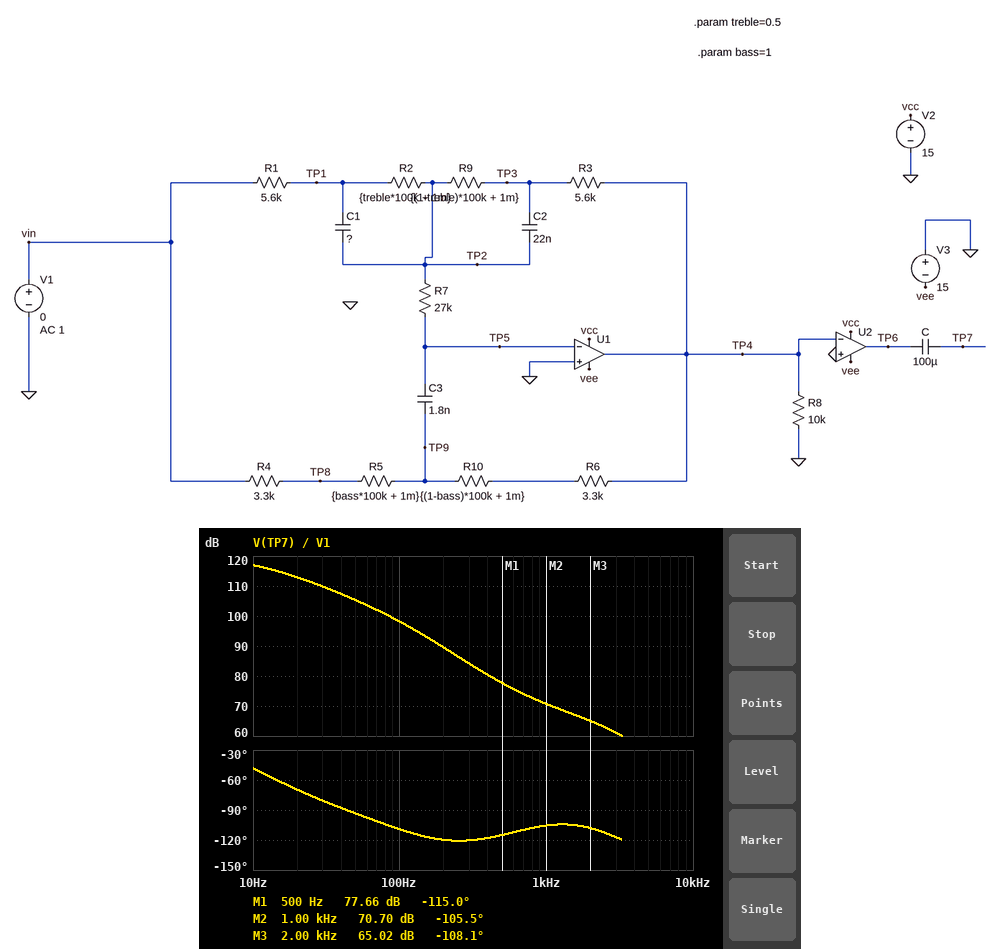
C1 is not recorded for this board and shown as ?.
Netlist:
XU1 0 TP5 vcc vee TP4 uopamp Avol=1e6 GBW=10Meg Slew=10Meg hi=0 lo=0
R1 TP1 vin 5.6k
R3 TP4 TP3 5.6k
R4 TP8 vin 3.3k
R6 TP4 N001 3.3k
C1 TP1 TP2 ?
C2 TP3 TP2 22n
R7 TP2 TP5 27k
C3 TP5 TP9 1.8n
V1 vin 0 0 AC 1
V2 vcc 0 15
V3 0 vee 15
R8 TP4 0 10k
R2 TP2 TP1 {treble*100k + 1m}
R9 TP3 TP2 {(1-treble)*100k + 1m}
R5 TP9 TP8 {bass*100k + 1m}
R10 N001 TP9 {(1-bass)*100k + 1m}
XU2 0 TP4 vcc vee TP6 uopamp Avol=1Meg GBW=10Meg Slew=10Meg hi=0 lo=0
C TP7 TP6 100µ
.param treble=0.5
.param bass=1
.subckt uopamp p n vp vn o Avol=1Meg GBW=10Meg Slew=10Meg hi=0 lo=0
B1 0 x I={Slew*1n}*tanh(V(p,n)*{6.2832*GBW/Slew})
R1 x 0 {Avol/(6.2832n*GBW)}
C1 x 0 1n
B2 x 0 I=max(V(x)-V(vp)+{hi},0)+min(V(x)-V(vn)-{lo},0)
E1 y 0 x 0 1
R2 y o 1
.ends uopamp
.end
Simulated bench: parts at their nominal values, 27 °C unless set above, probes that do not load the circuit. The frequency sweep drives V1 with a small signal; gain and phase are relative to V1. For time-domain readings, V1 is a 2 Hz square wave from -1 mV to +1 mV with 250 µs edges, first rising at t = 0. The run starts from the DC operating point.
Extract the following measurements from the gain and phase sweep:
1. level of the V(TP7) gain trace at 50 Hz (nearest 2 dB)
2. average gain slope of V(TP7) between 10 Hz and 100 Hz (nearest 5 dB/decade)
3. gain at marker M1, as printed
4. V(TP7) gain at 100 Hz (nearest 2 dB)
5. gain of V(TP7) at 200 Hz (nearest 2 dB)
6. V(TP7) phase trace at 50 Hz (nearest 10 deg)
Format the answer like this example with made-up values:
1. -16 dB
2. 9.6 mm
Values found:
1. 106 dB
2. -20 dB/decade
3. 77.66 dB
4. 98 dB
5. 90 dB
6. -90 deg
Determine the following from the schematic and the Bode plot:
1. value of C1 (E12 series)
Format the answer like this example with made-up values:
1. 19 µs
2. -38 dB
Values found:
1. 6.8 nF
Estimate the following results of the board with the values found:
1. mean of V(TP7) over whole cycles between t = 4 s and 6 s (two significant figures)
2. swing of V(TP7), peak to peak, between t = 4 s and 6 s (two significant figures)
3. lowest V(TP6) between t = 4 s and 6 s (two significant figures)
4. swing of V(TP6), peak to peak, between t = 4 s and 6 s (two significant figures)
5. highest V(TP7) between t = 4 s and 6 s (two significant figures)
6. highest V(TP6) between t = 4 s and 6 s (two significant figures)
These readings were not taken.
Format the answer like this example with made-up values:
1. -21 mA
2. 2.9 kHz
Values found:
1. 15 V
2. 30 V
3. -15 V
4. 30 V
5. 30 V
6. 15 V
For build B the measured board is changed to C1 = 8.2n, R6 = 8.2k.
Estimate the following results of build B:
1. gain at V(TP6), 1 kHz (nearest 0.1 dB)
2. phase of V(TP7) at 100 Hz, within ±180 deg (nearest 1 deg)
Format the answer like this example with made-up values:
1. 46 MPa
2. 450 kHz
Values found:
1. 72.1 dB
2. -107 deg
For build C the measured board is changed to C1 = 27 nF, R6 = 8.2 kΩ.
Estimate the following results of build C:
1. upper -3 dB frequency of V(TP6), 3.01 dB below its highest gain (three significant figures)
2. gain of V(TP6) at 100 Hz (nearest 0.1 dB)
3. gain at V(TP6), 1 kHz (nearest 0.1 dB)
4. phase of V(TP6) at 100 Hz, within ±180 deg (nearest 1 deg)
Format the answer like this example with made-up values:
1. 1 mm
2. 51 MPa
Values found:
1. 10.0 Hz
2. 100.4 dB
3. 78.7 dB
4. -85 deg
